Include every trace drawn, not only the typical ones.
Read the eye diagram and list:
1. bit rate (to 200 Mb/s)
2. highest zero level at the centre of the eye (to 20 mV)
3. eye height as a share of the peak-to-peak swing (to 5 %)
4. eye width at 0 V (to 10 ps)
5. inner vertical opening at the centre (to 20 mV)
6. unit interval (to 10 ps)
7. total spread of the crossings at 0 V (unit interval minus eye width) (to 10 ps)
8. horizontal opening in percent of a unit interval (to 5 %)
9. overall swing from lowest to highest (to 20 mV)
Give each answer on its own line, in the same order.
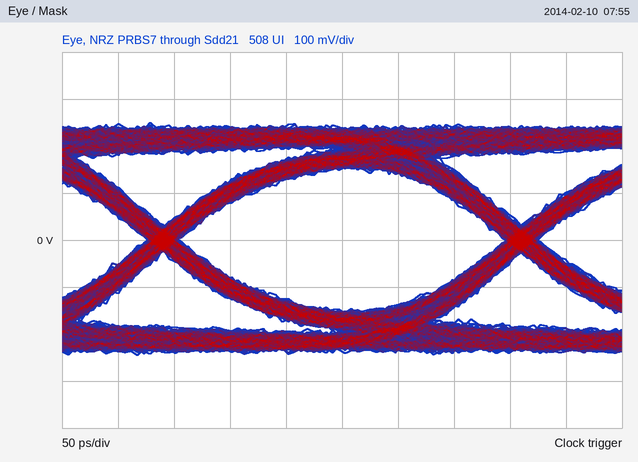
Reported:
3.2 Gb/s
-160 mV
60 %
290 ps
300 mV
320 ps
30 ps
90 %
500 mV
